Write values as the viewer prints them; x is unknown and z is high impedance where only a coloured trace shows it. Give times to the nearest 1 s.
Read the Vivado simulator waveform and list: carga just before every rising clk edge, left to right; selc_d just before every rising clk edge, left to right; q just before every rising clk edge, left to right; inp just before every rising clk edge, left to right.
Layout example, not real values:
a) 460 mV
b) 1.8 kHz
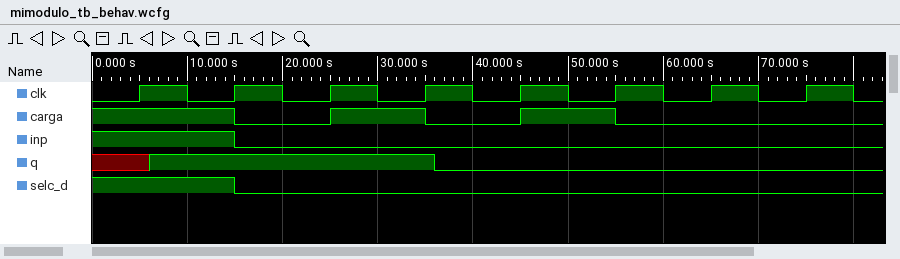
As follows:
a) 1 1 0 1 0 1 0 0
b) 1 1 0 0 0 0 0 0
c) x 1 1 1 0 0 0 0
d) 1 1 0 0 0 0 0 0
